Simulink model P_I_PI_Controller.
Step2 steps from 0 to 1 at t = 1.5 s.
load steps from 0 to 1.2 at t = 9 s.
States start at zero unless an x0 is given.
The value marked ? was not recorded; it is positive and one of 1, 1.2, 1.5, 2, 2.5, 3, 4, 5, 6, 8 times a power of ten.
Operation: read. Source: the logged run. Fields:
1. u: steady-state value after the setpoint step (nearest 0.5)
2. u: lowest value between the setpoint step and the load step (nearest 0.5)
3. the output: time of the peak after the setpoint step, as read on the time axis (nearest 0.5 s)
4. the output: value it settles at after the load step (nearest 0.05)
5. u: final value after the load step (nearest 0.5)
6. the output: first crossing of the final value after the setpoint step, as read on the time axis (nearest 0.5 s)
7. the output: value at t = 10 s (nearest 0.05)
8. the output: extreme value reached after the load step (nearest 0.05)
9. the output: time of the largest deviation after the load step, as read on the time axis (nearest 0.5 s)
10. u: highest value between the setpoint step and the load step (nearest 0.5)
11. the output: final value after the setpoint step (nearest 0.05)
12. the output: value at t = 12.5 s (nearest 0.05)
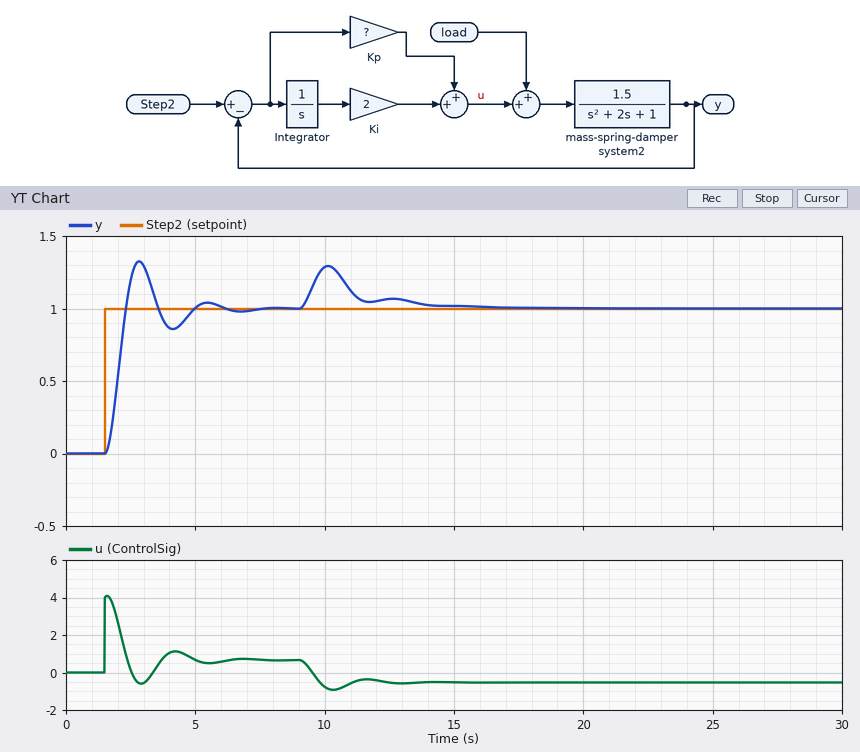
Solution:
0.5
-0.5
3.0 s
1.00
-0.5
2.5 s
1.30
1.30
10.0 s
4.0
1.00
1.05
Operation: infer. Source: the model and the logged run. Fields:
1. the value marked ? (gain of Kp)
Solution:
4
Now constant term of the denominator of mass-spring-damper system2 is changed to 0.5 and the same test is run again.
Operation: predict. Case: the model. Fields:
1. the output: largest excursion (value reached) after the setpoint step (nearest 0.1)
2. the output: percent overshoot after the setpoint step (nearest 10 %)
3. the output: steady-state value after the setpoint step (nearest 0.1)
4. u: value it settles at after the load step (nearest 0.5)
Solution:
1.4
40 %
1.0
-1.0
